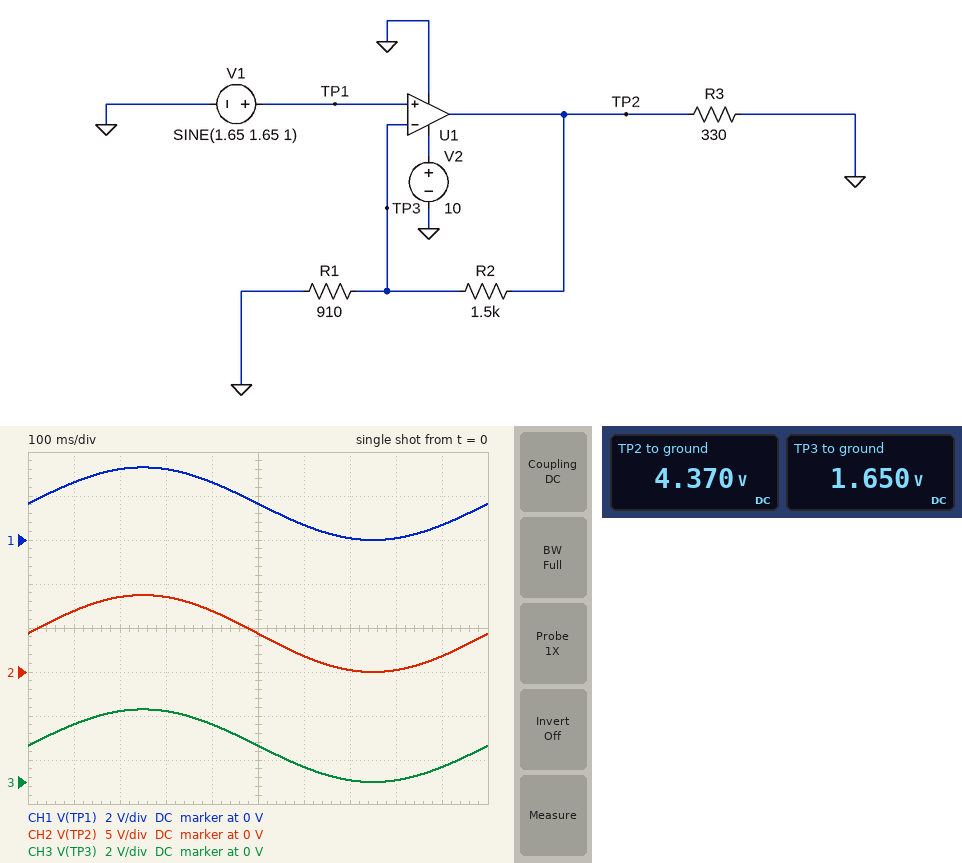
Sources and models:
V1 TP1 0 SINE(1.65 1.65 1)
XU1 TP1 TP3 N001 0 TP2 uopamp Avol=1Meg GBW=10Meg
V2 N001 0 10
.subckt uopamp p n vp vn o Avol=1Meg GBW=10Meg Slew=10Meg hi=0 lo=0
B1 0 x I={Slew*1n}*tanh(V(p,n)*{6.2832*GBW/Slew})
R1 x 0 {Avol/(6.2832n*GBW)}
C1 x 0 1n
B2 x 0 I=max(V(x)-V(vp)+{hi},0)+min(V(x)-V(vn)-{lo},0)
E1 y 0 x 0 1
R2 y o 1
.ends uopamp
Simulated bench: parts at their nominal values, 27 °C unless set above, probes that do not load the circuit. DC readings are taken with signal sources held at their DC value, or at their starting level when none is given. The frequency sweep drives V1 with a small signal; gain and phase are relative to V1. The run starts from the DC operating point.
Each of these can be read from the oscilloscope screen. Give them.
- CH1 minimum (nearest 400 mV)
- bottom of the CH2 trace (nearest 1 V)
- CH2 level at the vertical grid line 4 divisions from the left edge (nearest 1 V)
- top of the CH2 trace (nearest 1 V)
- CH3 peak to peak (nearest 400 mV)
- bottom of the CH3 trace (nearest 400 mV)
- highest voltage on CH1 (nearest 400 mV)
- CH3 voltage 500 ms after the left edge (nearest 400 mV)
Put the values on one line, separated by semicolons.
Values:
0 V; 0 V; 7 V; 9 V; 3.2 V; 0 V; 3.2 V; 1.6 V
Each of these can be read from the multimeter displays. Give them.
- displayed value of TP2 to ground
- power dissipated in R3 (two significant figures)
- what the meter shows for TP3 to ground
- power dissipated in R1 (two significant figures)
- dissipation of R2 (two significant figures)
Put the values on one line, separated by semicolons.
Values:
4.370 V; 58 mW; 1.650 V; 3.0 mW; 4.9 mW
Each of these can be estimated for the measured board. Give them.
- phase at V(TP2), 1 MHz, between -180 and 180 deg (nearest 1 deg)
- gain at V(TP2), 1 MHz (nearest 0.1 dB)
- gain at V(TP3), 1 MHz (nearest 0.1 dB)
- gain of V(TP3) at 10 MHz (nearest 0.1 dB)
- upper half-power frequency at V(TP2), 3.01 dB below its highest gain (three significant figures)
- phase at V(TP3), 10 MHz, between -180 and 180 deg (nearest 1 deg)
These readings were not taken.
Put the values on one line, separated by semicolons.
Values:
-15 deg; 8.2 dB; -0.3 dB; -9.1 dB; 3.76 MHz; -69 deg
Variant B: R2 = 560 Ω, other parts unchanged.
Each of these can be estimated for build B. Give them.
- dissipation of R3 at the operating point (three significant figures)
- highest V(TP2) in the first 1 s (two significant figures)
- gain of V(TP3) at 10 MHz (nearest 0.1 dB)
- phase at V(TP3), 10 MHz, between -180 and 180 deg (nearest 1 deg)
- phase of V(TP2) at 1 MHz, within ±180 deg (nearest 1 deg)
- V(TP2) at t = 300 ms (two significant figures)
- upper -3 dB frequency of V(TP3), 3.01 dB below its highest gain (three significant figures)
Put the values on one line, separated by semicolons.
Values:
21.5 mW; 5.3 V; -5.6 dB; -58 deg; -9 deg; 5.2 V; 6.17 MHz
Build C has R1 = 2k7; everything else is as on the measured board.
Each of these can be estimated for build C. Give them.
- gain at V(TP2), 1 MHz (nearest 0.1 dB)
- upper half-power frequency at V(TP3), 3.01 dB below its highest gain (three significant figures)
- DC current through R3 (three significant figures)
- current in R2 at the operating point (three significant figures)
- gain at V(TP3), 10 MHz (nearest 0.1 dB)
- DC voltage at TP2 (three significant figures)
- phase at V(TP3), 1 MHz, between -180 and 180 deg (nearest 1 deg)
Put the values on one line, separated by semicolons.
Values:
3.7 dB; 6.41 MHz; 7.78 mA; 611 µA; -5.4 dB; 2.57 V; -9 deg
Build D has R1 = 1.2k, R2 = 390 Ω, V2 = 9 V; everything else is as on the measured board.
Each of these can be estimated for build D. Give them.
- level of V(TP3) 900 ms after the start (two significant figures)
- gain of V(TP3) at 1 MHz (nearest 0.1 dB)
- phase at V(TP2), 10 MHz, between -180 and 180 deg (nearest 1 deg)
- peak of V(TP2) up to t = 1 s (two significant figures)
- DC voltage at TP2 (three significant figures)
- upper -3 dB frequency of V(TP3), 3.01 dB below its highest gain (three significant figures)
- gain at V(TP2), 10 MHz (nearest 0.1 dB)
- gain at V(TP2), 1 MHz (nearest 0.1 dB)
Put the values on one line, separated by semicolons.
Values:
680 mV; -0.1 dB; -53 deg; 4.4 V; 2.19 V; 7.52 MHz; -2.0 dB; 2.4 dB
